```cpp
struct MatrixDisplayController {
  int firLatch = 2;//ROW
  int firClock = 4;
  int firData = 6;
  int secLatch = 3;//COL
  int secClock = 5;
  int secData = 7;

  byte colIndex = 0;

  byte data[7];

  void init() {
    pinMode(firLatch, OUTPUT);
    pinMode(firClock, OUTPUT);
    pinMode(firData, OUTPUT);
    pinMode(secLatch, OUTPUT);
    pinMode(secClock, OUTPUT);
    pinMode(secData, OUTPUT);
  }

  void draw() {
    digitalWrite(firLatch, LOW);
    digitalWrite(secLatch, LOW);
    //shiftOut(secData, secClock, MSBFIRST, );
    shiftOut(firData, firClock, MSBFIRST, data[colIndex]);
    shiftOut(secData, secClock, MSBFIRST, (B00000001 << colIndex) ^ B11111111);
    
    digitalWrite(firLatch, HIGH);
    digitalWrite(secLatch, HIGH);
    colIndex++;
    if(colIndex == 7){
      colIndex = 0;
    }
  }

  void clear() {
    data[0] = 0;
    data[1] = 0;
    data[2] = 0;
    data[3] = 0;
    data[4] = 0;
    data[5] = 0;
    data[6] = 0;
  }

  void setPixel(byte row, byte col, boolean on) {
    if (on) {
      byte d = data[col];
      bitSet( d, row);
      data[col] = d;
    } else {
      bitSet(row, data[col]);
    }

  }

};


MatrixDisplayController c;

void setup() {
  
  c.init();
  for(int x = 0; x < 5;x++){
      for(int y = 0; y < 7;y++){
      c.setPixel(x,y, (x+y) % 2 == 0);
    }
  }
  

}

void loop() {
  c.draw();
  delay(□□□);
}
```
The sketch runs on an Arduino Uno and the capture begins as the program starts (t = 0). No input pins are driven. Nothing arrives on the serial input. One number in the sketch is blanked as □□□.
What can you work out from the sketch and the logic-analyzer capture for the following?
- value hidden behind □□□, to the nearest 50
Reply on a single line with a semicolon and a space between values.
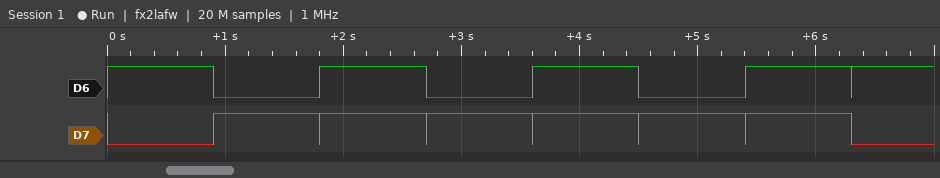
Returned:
900
